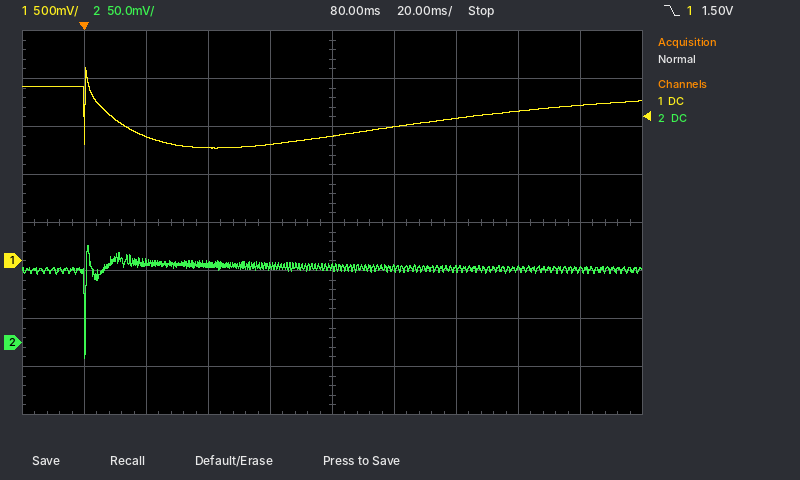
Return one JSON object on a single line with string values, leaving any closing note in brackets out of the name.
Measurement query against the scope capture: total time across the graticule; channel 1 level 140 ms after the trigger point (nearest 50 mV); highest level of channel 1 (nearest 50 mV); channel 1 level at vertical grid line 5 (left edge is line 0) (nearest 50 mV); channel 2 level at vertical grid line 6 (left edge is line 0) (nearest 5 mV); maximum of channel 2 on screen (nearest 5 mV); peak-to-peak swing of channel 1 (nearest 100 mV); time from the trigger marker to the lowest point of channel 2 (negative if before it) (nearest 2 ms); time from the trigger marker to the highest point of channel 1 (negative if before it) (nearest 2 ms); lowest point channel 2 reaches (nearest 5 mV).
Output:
{"total time across the graticule": "200 ms", "channel 1 level 140 ms after the trigger point": "1.55 V", "highest level of channel 1": "2.00 V", "channel 1 level at vertical grid line 5 (left edge is line 0)": "1.30 V", "channel 2 level at vertical grid line 6 (left edge is line 0)": "75 mV", "maximum of channel 2 on screen": "100 mV", "peak-to-peak swing of channel 1": "800 mV", "time from the trigger marker to the lowest point of channel 2 (negative if before it)": "0 ms", "time from the trigger marker to the highest point of channel 1 (negative if before it)": "0 ms", "lowest point channel 2 reaches": "-15 mV"}
